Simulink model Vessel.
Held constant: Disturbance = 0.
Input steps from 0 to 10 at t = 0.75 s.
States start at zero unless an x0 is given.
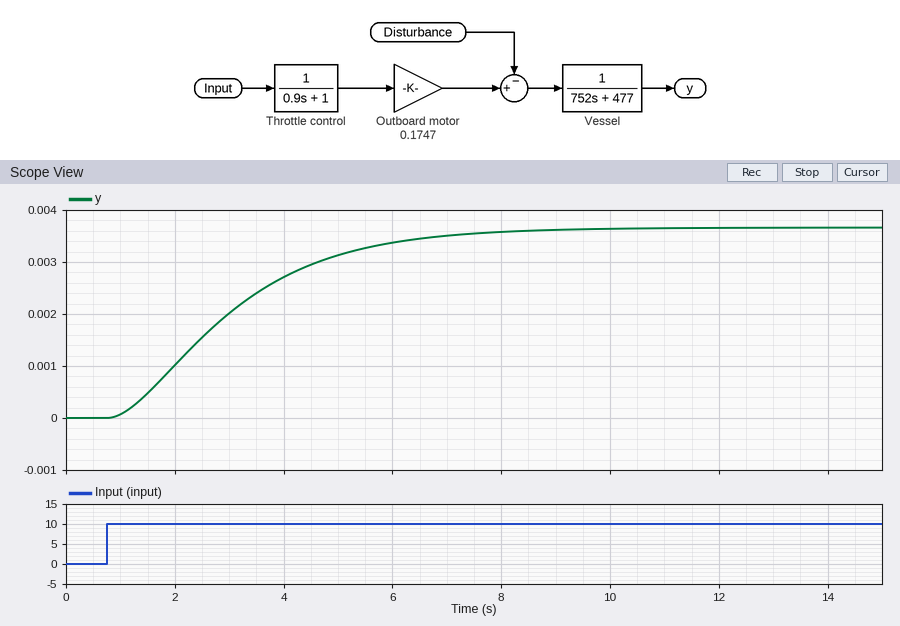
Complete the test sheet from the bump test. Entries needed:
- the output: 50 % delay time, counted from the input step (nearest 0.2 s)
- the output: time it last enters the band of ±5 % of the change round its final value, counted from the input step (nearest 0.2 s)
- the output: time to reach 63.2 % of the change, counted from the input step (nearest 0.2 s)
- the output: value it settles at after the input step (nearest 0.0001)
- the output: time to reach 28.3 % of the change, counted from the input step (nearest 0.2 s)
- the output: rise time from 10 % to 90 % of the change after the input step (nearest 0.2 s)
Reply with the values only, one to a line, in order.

2.0 s
6.0 s
2.6 s
0.0037
1.2 s
4.2 s
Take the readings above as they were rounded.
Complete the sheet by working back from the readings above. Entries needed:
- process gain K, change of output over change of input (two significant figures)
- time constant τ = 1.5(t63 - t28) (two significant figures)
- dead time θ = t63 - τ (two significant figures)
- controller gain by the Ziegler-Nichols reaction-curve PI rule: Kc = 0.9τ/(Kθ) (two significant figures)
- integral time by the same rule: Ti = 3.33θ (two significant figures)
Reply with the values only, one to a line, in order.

0.00037
2.1 s
0.50 s
10000
1.7 s
